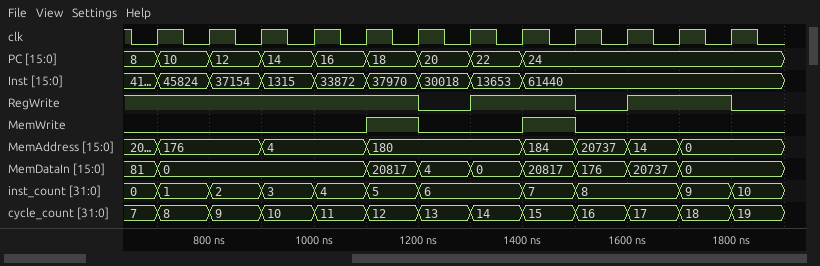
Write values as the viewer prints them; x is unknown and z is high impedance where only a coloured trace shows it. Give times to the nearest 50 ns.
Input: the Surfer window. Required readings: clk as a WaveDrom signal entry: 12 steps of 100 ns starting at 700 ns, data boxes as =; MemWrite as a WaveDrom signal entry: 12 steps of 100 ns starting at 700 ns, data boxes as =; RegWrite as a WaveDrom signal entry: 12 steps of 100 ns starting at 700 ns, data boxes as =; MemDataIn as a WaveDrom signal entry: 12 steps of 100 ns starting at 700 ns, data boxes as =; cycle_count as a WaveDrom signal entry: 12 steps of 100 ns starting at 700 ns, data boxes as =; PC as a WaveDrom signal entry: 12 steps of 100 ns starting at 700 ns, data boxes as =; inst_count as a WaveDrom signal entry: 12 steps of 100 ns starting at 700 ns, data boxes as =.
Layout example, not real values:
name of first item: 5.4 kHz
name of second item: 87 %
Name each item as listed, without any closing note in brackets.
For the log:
clk as a WaveDrom signal entry: 12 steps of 100 ns starting at 700 ns, data boxes as =: {name: 'clk', wave: 'p...........'}
MemWrite as a WaveDrom signal entry: 12 steps of 100 ns starting at 700 ns, data boxes as =: {name: 'MemWrite', wave: '0...10.10...'}
RegWrite as a WaveDrom signal entry: 12 steps of 100 ns starting at 700 ns, data boxes as =: {name: 'RegWrite', wave: '1....01.01.0'}
MemDataIn as a WaveDrom signal entry: 12 steps of 100 ns starting at 700 ns, data boxes as =: {name: 'MemDataIn', wave: '=...=======.', data: '0 20817 4 0 20817 176 20737 0'}
cycle_count as a WaveDrom signal entry: 12 steps of 100 ns starting at 700 ns, data boxes as =: {name: 'cycle_count', wave: '============', data: '8 9 10 11 12 13 14 15 16 17 18 19'}
PC as a WaveDrom signal entry: 12 steps of 100 ns starting at 700 ns, data boxes as =: {name: 'PC', wave: '========....', data: '10 12 14 16 18 20 22 24'}
inst_count as a WaveDrom signal entry: 12 steps of 100 ns starting at 700 ns, data boxes as =: {name: 'inst_count', wave: '======.==.==', data: '1 2 3 4 5 6 7 8 9 10'}
